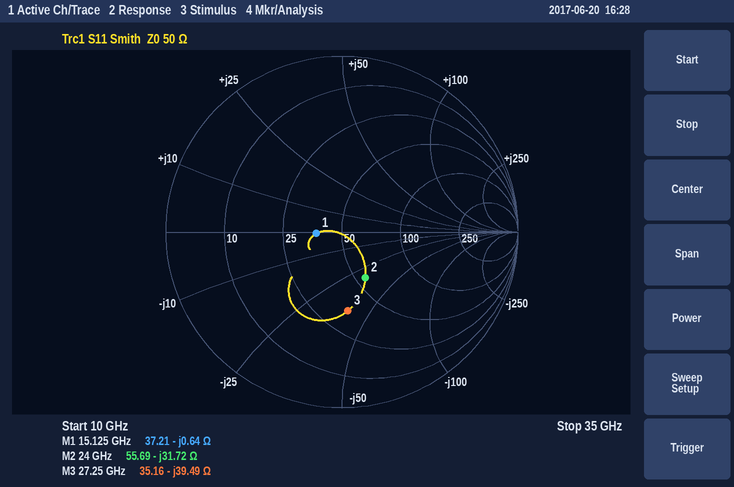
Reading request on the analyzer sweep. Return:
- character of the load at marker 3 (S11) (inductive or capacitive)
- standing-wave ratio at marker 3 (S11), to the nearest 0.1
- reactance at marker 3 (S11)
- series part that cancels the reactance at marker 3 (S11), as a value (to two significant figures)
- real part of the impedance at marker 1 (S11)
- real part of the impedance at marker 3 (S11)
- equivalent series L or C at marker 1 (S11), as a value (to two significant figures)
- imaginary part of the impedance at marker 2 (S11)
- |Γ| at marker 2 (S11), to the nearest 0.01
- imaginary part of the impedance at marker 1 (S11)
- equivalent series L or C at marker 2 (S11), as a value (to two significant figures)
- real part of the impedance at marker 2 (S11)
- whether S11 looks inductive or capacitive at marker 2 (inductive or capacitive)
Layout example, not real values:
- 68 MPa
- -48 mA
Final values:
- capacitive
- 2.6
- -39.49 Ω
- 230 pH
- 37.21 Ω
- 35.16 Ω
- 16 pF
- -31.72 Ω
- 0.29
- -0.64 Ω
- 210 fF
- 55.69 Ω
- capacitive
